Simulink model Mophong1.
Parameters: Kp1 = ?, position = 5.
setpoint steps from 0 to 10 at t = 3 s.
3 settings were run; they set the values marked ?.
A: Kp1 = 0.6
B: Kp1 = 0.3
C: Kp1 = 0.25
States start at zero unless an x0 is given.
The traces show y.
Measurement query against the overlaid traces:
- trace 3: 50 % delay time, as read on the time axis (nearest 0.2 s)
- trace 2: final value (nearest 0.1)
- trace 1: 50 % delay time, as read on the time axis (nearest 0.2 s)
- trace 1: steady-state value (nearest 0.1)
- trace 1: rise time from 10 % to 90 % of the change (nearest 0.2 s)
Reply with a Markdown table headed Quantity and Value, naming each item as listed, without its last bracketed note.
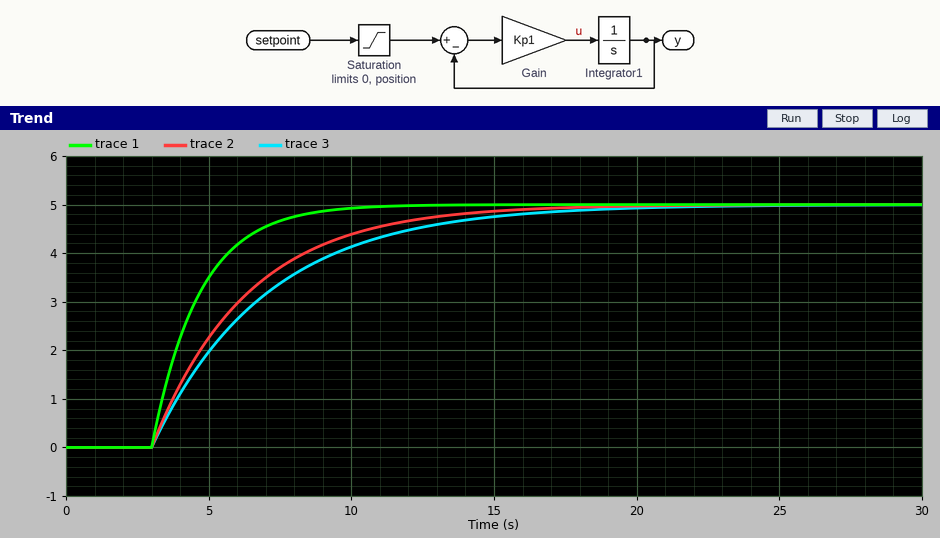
| Quantity | Value |
|---|---|
| trace 3: 50 % delay time, as read on the time axis | 5.8 s |
| trace 2: final value | 5.0 |
| trace 1: 50 % delay time, as read on the time axis | 4.2 s |
| trace 1: steady-state value | 5.0 |
| trace 1: rise time from 10 % to 90 % of the change | 3.6 s |
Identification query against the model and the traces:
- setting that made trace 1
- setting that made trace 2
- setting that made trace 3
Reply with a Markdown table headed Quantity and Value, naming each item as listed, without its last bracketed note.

| Quantity | Value |
|---|---|
| setting that made trace 1 | A |
| setting that made trace 2 | B |
| setting that made trace 3 | C |
